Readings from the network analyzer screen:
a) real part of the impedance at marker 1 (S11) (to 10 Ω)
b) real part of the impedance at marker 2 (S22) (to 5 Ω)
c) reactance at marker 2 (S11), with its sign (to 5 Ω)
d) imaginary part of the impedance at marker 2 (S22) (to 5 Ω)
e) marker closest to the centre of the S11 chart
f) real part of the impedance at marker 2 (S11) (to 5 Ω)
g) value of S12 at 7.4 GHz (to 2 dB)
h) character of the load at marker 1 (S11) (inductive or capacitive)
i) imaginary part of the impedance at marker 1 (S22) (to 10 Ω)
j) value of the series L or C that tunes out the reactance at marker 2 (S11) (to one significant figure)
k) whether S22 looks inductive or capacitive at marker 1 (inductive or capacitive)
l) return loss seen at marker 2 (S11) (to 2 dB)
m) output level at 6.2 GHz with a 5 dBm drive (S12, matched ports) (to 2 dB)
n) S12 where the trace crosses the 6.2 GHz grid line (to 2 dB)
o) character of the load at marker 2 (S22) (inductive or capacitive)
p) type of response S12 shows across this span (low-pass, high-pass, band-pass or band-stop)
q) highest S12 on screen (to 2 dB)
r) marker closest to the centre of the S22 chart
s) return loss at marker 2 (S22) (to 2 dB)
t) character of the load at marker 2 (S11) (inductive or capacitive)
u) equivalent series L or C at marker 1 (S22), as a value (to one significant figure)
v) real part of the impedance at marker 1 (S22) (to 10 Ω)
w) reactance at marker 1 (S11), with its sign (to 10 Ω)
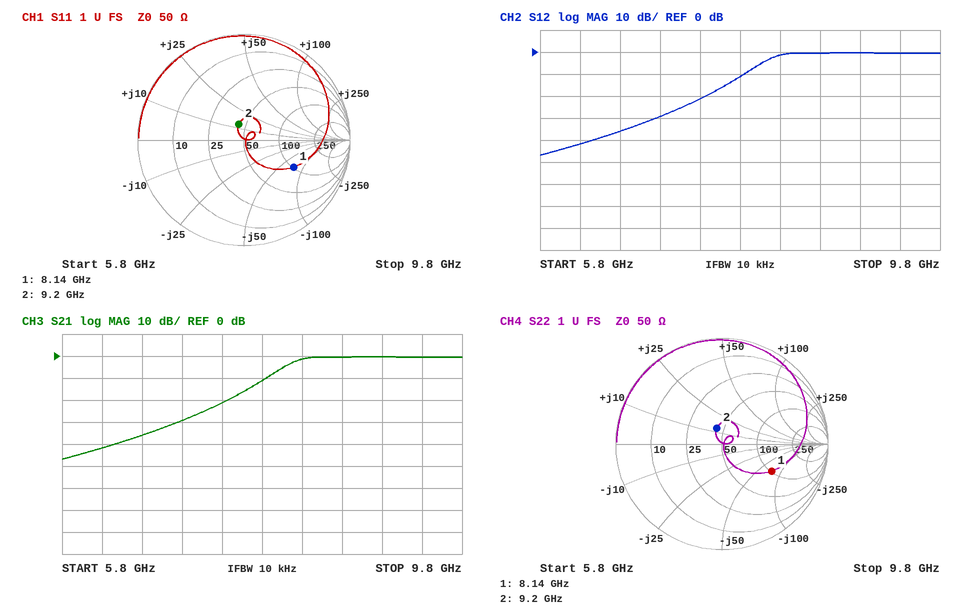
100 Ω
45 Ω
+15 Ω
+15 Ω
marker 2
45 Ω
-22 dB
capacitive
-70 Ω
1 pF
capacitive
16 dB
-36 dBm
-42 dB
inductive
high-pass
0 dB
marker 2
16 dB
inductive
300 fF
100 Ω
-70 Ω
